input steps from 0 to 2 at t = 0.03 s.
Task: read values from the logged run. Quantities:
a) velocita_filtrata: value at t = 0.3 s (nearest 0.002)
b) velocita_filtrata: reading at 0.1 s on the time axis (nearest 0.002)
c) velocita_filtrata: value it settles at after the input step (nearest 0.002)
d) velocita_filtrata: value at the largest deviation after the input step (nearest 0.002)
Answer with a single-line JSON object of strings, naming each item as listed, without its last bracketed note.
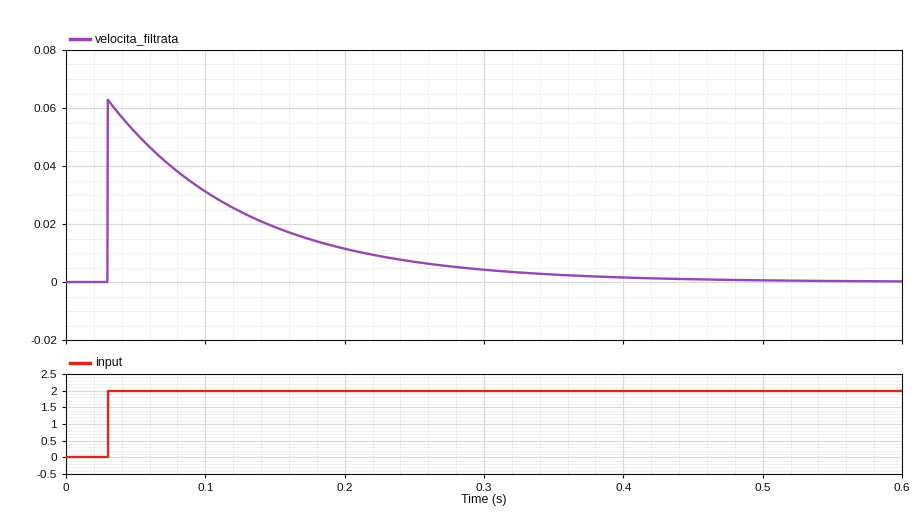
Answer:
{"velocita_filtrata: value at t = 0.3 s": "0.004", "velocita_filtrata: reading at 0.1 s on the time axis": "0.032", "velocita_filtrata: value it settles at after the input step": "0.000", "velocita_filtrata: value at the largest deviation after the input step": "0.062"}
